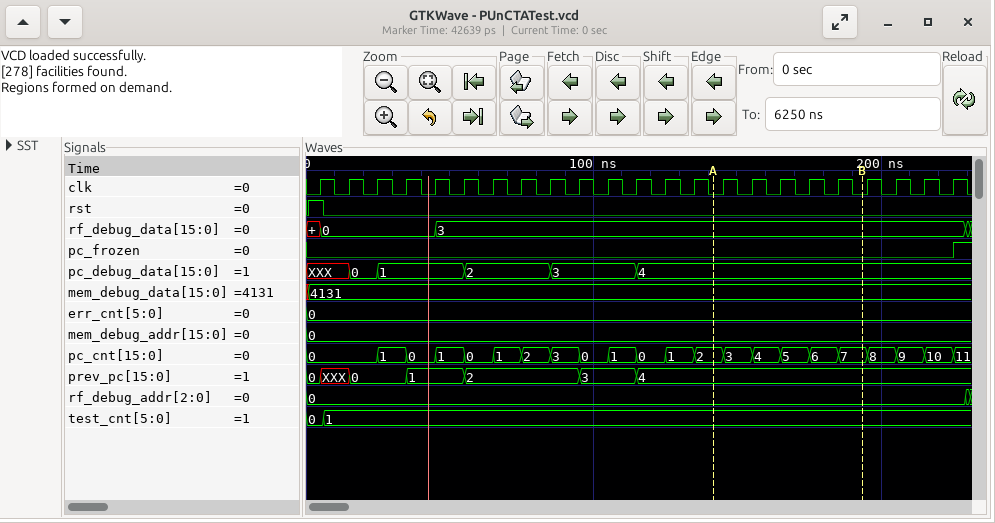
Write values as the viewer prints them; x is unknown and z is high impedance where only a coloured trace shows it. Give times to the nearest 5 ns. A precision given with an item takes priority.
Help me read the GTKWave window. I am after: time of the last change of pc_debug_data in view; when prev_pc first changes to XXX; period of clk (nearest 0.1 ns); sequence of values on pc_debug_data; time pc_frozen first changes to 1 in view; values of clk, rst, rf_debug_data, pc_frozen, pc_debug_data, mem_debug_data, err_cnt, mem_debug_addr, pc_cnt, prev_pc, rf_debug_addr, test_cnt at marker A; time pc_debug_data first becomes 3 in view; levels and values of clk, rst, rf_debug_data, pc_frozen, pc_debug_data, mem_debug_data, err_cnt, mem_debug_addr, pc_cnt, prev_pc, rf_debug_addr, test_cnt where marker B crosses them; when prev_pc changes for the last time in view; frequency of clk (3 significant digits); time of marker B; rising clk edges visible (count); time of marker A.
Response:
115 ns
5 ns
10 ns
XXX, 0, 1, 2, 3, 4
225 ns
clk=0, rst=0, rf_debug_data=3, pc_frozen=0, pc_debug_data=4, mem_debug_data=4131, err_cnt=0, mem_debug_addr=0, pc_cnt=2, prev_pc=4, rf_debug_addr=0, test_cnt=1
85 ns
clk=0, rst=0, rf_debug_data=3, pc_frozen=0, pc_debug_data=4, mem_debug_data=4131, err_cnt=0, mem_debug_addr=0, pc_cnt=7, prev_pc=4, rf_debug_addr=0, test_cnt=1
115 ns
100 MHz
195 ns
23
140 ns
